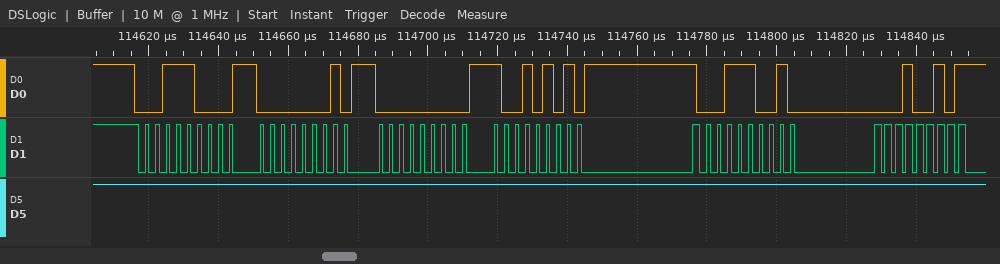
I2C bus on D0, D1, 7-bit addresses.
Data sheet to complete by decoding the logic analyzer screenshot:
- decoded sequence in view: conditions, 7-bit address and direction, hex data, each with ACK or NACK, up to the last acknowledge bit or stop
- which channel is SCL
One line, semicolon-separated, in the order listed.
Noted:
start, address 1C write ACK, 01 ACK, 00 ACK, 95 ACK, repeated start, address 1C read ACK, 12 NACK; D1
